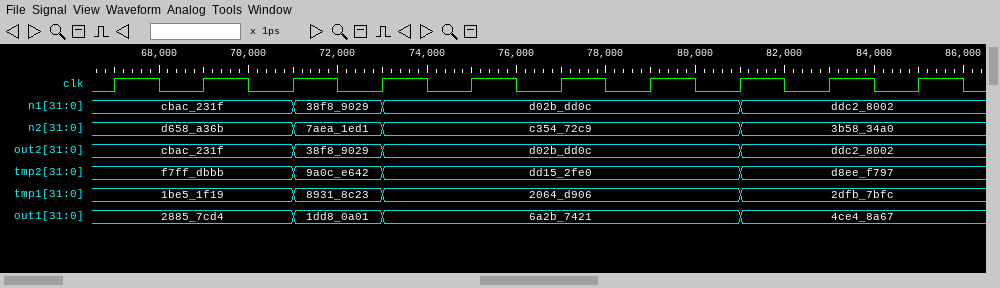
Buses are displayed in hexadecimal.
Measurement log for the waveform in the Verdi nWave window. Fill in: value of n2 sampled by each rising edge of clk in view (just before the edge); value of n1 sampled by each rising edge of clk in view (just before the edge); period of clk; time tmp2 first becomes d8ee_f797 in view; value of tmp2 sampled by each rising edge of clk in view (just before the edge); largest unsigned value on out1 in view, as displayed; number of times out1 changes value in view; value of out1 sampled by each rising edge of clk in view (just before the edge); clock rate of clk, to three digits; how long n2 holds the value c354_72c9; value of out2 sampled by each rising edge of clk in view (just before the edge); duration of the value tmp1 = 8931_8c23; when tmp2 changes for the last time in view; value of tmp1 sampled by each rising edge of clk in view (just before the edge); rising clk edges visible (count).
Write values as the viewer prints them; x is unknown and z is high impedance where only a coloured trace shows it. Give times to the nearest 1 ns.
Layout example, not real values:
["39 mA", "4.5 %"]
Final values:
["d658_a36b, d658_a36b, d658_a36b, 7aea_1ed1, c354_72c9, c354_72c9, c354_72c9, c354_72c9, 3b58_34a0, 3b58_34a0", "cbac_231f, cbac_231f, cbac_231f, 38f8_9029, d02b_dd0c, d02b_dd0c, d02b_dd0c, d02b_dd0c, ddc2_8002, ddc2_8002", "2 ns", "81 ns", "f7ff_dbbb, f7ff_dbbb, f7ff_dbbb, 9a0c_e642, dd15_2fe0, dd15_2fe0, dd15_2fe0, dd15_2fe0, d8ee_f797, d8ee_f797", "6a2b_7421", "3", "2885_7cd4, 2885_7cd4, 2885_7cd4, 1dd8_0a01, 6a2b_7421, 6a2b_7421, 6a2b_7421, 6a2b_7421, 4ce4_8a67, 4ce4_8a67", "500 MHz", "8 ns", "cbac_231f, cbac_231f, cbac_231f, 38f8_9029, d02b_dd0c, d02b_dd0c, d02b_dd0c, d02b_dd0c, ddc2_8002, ddc2_8002", "2 ns", "81 ns", "1be5_1f19, 1be5_1f19, 1be5_1f19, 8931_8c23, 2064_d906, 2064_d906, 2064_d906, 2064_d906, 2dfb_7bfc, 2dfb_7bfc", "10"]
